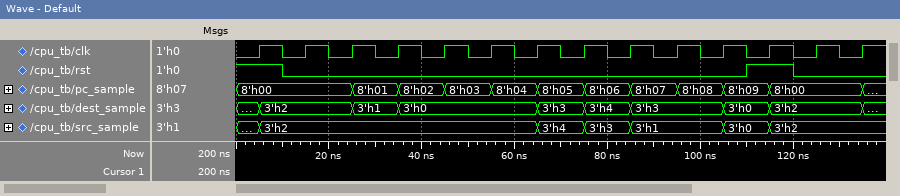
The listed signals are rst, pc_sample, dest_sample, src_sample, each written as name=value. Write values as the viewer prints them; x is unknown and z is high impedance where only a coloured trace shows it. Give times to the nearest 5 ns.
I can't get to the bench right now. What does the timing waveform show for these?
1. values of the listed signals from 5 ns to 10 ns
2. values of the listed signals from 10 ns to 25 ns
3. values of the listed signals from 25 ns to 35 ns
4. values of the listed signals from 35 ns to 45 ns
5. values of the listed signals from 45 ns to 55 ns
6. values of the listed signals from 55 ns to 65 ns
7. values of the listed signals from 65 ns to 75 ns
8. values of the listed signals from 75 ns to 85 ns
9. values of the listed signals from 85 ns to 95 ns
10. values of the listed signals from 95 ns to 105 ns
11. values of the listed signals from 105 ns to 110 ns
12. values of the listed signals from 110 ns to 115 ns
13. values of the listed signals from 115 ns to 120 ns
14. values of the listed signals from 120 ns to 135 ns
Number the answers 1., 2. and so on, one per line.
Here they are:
1. rst=1, pc_sample=8'h00, dest_sample=3'h2, src_sample=3'h2
2. rst=0, pc_sample=8'h00, dest_sample=3'h2, src_sample=3'h2
3. rst=0, pc_sample=8'h01, dest_sample=3'h1, src_sample=3'h2
4. rst=0, pc_sample=8'h02, dest_sample=3'h0, src_sample=3'h2
5. rst=0, pc_sample=8'h03, dest_sample=3'h0, src_sample=3'h2
6. rst=0, pc_sample=8'h04, dest_sample=3'h0, src_sample=3'h2
7. rst=0, pc_sample=8'h05, dest_sample=3'h3, src_sample=3'h4
8. rst=0, pc_sample=8'h06, dest_sample=3'h4, src_sample=3'h3
9. rst=0, pc_sample=8'h07, dest_sample=3'h3, src_sample=3'h1
10. rst=0, pc_sample=8'h08, dest_sample=3'h3, src_sample=3'h1
11. rst=0, pc_sample=8'h09, dest_sample=3'h0, src_sample=3'h0
12. rst=1, pc_sample=8'h09, dest_sample=3'h0, src_sample=3'h0
13. rst=1, pc_sample=8'h00, dest_sample=3'h2, src_sample=3'h2
14. rst=0, pc_sample=8'h00, dest_sample=3'h2, src_sample=3'h2
